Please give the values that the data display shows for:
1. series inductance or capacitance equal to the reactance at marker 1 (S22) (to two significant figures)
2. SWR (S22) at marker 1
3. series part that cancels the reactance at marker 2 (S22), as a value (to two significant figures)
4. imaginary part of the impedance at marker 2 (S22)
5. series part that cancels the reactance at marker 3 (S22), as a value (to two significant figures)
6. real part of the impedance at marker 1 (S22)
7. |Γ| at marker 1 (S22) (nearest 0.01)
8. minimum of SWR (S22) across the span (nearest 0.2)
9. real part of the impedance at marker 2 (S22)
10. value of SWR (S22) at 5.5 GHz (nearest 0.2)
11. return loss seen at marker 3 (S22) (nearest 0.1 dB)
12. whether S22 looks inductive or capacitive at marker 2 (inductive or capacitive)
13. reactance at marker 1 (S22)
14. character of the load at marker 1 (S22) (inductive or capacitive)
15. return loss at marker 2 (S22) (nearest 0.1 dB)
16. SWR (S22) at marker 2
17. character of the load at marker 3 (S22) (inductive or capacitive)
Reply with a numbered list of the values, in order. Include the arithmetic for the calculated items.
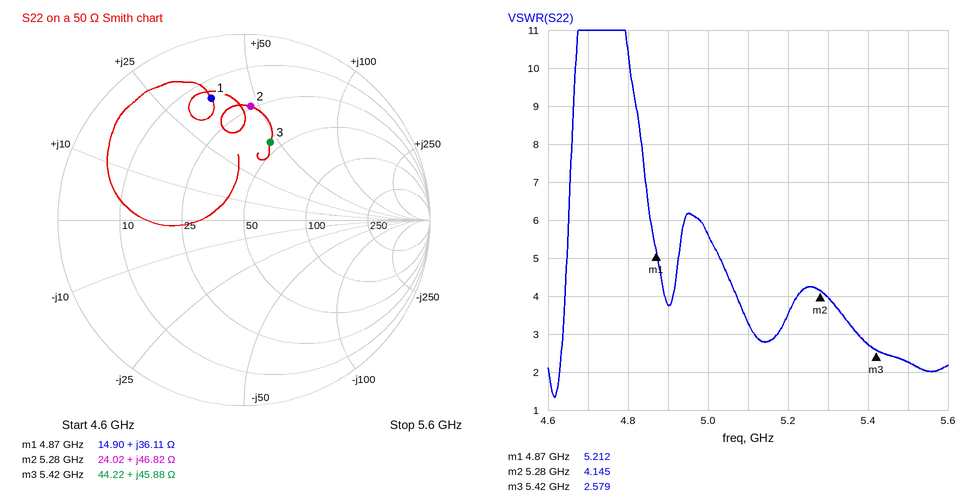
1. L = 36.11 Ω/(2π × 4.87 GHz) ≈ 1.2 nH
2. 5.212
3. C = 1/(2π × 5.28 GHz × 46.82 Ω) ≈ 644 fF, so 640 fF to two significant figures
4. +46.82 Ω
5. C = 1/(2π × 5.42 GHz × 45.88 Ω) ≈ 640 fF
6. 14.90 Ω
7. 0.68
8. 1.4
9. 24.02 Ω
10. 2.2
11. 7.1 dB
12. inductive
13. +36.11 Ω
14. inductive
15. 4.3 dB
16. 4.145
17. inductive
